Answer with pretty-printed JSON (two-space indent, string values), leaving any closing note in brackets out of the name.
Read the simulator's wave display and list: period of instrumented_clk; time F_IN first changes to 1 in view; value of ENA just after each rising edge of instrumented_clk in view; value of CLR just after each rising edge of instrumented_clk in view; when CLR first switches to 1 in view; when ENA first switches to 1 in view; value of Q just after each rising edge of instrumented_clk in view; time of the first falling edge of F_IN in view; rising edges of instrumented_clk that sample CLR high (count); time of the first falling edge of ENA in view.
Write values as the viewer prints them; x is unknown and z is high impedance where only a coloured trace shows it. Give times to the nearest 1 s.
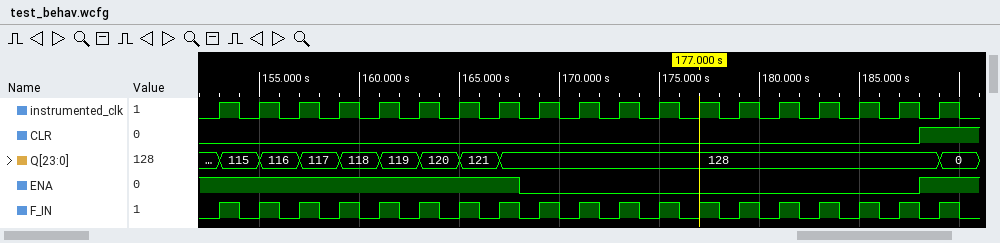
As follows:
{
  "period of instrumented_clk": "2 s",
  "time F_IN first changes to 1 in view": "153 s",
  "value of ENA just after each rising edge of instrumented_clk in view": "1 1 1 1 1 1 1 1 0 0 0 0 0 0 0 0 0 0 1",
  "value of CLR just after each rising edge of instrumented_clk in view": "0 0 0 0 0 0 0 0 0 0 0 0 0 0 0 0 0 0 1",
  "when CLR first switches to 1 in view": "188 s",
  "when ENA first switches to 1 in view": "188 s",
  "value of Q just after each rising edge of instrumented_clk in view": "115, 116, 117, 118, 119, 120, 121, 128, 128, 128, 128, 128, 128, 128, 128, 128, 128, 128, 0",
  "time of the first falling edge of F_IN in view": "154 s",
  "rising edges of instrumented_clk that sample CLR high": "1",
  "time of the first falling edge of ENA in view": "168 s"
}
